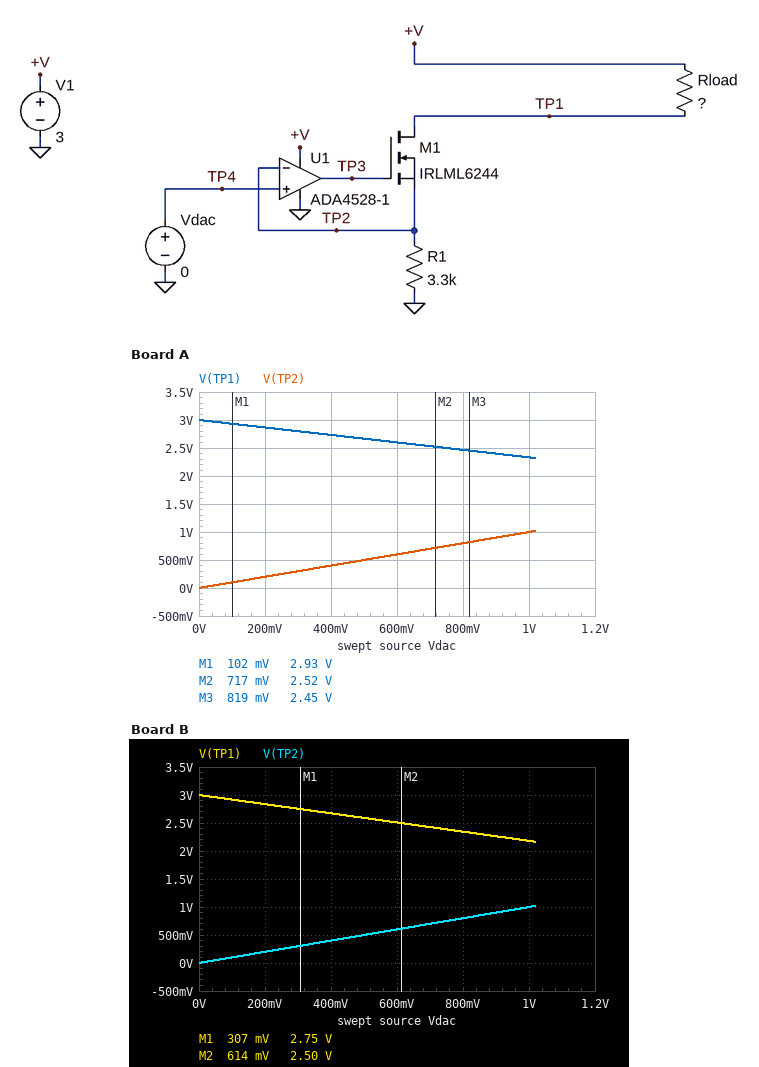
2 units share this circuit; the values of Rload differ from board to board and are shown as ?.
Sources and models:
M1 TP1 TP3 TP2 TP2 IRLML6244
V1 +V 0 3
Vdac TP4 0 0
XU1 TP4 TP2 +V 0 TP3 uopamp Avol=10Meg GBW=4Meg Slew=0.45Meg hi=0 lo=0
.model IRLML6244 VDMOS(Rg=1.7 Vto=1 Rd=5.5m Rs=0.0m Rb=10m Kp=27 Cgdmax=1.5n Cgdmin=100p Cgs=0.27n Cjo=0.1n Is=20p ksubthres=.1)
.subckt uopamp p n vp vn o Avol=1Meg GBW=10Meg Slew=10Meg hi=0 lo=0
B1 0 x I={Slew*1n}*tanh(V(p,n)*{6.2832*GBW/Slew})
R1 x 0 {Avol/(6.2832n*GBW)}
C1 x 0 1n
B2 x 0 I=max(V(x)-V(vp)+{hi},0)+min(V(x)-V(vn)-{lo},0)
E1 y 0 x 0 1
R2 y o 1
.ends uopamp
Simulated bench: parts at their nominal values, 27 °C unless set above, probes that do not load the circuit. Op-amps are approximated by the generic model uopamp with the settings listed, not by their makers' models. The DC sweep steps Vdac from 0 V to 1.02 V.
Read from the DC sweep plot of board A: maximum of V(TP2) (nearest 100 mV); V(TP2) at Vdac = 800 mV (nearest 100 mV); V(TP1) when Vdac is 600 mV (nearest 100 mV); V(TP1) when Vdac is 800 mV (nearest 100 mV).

1.0 V
800 mV
2.6 V
2.5 V
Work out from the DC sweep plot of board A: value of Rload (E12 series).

2.2 kΩ
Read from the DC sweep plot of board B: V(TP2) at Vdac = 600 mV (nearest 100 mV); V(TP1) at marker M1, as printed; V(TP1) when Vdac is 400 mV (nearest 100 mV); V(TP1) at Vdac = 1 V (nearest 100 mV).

600 mV
2.75 V
2.7 V
2.2 V
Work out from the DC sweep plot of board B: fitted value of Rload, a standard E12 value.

2.7 kΩ
